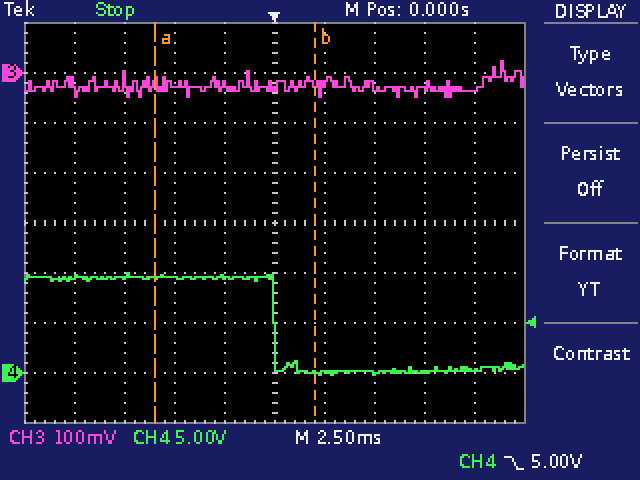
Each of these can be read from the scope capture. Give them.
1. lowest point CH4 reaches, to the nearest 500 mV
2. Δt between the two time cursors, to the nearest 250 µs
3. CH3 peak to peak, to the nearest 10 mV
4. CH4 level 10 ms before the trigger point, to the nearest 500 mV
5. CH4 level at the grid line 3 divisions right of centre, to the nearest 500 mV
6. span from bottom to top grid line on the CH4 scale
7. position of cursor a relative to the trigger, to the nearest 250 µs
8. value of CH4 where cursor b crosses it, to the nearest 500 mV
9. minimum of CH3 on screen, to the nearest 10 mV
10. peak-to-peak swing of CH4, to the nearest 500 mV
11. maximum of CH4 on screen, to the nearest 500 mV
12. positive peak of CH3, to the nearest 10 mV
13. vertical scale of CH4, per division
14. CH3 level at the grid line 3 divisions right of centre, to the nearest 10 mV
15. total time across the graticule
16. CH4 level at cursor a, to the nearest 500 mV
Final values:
0.0 V
8.00 ms
70 mV
9.5 V
0.0 V
40 V
-6.00 ms
0.0 V
-50 mV
10.0 V
10.0 V
20 mV
5 V
-30 mV
25 ms
9.5 V
